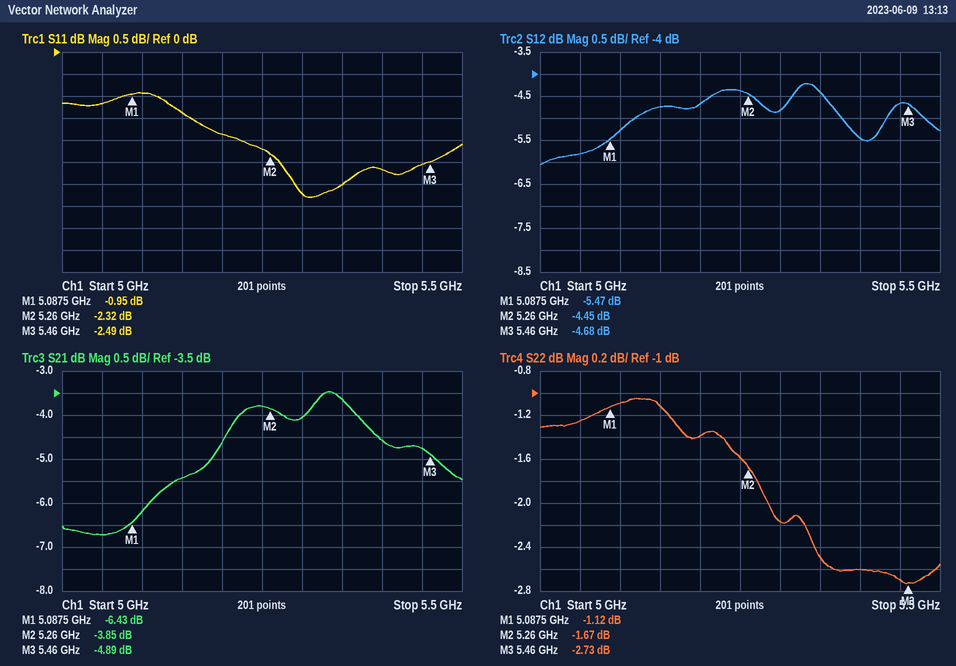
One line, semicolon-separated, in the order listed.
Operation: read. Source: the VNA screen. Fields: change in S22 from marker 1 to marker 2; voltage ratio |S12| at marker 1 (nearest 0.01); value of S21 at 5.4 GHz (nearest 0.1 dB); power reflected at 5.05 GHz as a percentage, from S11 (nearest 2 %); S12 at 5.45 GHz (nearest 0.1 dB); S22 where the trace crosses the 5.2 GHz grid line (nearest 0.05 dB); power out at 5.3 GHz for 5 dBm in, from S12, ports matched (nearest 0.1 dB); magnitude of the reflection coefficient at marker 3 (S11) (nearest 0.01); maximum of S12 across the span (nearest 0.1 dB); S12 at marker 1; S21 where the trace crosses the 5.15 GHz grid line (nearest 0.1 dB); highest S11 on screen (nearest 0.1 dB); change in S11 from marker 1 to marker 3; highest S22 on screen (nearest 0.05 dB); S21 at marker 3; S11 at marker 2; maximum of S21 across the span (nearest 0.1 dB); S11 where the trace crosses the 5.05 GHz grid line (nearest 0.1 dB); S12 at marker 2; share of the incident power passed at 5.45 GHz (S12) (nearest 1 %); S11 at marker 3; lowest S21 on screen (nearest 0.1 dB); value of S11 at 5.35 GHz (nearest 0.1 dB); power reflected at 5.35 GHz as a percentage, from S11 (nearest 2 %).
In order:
-0.55 dB; 0.53; -4.6 dB; 76 %; -4.7 dB; -1.40 dB; 0.2 dBm; 0.75; -4.2 dB; -5.47 dB; -5.4 dB; -0.9 dB; -1.54 dB; -1.05 dB; -4.89 dB; -2.32 dB; -3.5 dB; -1.2 dB; -4.45 dB; 34 %; -2.49 dB; -6.7 dB; -3.0 dB; 50 %
